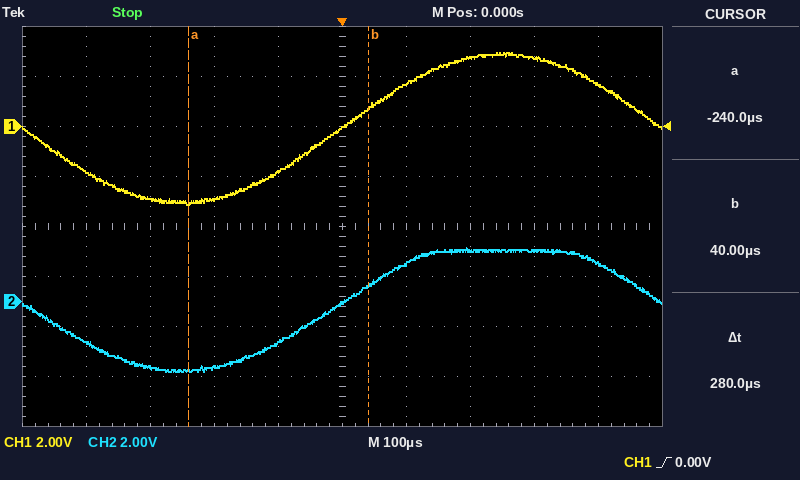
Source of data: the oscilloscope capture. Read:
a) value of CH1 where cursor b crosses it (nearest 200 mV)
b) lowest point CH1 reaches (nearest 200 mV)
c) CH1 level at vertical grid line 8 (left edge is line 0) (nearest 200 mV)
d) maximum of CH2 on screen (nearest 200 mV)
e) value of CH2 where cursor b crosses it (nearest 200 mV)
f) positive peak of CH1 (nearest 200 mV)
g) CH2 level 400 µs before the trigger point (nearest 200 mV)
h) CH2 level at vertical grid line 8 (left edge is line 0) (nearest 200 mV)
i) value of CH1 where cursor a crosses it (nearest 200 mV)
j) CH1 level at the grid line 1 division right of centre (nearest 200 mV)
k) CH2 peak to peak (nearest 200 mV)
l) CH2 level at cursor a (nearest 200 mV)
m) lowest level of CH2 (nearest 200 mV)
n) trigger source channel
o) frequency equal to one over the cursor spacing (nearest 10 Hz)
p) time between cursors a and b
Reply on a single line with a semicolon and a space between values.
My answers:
800 mV; -3.2 V; 2.8 V; 2.2 V; 600 mV; 3.0 V; -1.6 V; 2.0 V; -3.0 V; 1.8 V; 5.0 V; -2.8 V; -2.8 V; CH1; 3.57 kHz; 280 µs
